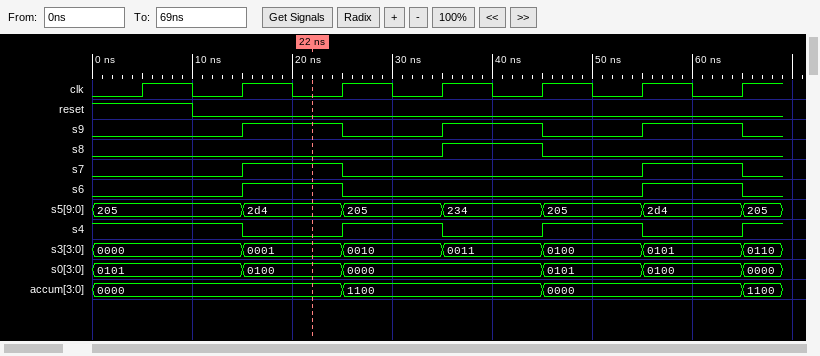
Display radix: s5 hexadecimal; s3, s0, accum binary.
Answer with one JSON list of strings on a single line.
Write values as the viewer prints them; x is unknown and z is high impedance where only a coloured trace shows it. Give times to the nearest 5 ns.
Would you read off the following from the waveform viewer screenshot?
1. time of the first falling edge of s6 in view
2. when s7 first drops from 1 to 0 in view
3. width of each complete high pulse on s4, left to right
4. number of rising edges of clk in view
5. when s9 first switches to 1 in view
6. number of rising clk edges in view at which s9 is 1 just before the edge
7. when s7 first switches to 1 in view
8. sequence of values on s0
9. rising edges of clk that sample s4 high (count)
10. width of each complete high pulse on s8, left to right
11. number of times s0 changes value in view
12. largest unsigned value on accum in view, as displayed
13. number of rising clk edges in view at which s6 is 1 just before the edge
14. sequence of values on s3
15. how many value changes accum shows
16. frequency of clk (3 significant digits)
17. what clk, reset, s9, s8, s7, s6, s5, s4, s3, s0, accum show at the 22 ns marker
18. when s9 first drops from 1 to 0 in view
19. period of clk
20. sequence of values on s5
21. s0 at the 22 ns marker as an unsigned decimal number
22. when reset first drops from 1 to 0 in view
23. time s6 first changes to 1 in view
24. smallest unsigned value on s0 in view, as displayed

["25 ns", "25 ns", "10 ns, 10 ns", "7", "15 ns", "3", "15 ns", "0101, 0100, 0000, 0101, 0100, 0000", "4", "10 ns", "5", "1100", "2", "0000, 0001, 0010, 0011, 0100, 0101, 0110", "3", "100 MHz", "clk=0, reset=0, s9=1, s8=0, s7=1, s6=1, s5=2d4, s4=0, s3=0001, s0=0100, accum=0000", "25 ns", "10 ns", "205, 2d4, 205, 234, 205, 2d4, 205", "4", "10 ns", "15 ns", "0000"]
